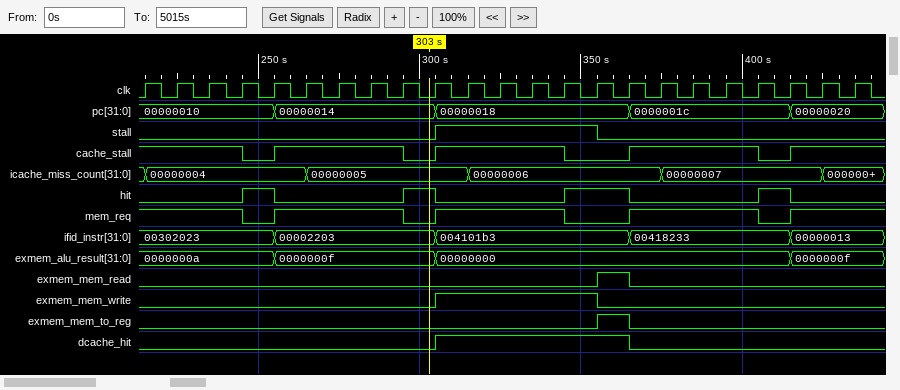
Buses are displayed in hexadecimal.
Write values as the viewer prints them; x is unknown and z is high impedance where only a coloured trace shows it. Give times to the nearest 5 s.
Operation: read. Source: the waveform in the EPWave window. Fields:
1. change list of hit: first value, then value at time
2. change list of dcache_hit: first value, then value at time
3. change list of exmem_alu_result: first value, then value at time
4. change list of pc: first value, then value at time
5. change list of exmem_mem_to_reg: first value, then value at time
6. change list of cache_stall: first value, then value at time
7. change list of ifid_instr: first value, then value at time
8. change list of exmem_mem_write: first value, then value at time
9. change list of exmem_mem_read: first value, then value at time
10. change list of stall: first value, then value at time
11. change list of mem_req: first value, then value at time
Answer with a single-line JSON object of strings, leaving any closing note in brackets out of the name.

{"change list of hit: first value, then value at time": "0, 1 at 245 s, 0 at 255 s, 1 at 295 s, 0 at 305 s, 1 at 345 s, 0 at 365 s, 1 at 405 s, 0 at 415 s", "change list of dcache_hit: first value, then value at time": "0, 1 at 305 s, 0 at 365 s", "change list of exmem_alu_result: first value, then value at time": "0000000a, 0000000f at 255 s, 00000000 at 305 s, 0000000f at 415 s", "change list of pc: first value, then value at time": "00000010, 00000014 at 255 s, 00000018 at 305 s, 0000001c at 365 s, 00000020 at 415 s", "change list of exmem_mem_to_reg: first value, then value at time": "0, 1 at 355 s, 0 at 365 s", "change list of cache_stall: first value, then value at time": "1, 0 at 245 s, 1 at 255 s, 0 at 295 s, 1 at 305 s, 0 at 345 s, 1 at 365 s, 0 at 405 s, 1 at 415 s", "change list of ifid_instr: first value, then value at time": "00302023, 00002203 at 255 s, 004101b3 at 305 s, 00418233 at 365 s, 00000013 at 415 s", "change list of exmem_mem_write: first value, then value at time": "0, 1 at 305 s, 0 at 355 s", "change list of exmem_mem_read: first value, then value at time": "0, 1 at 355 s, 0 at 365 s", "change list of stall: first value, then value at time": "0, 1 at 305 s, 0 at 355 s", "change list of mem_req: first value, then value at time": "1, 0 at 245 s, 1 at 255 s, 0 at 295 s, 1 at 305 s, 0 at 345 s, 1 at 365 s, 0 at 405 s, 1 at 415 s"}
